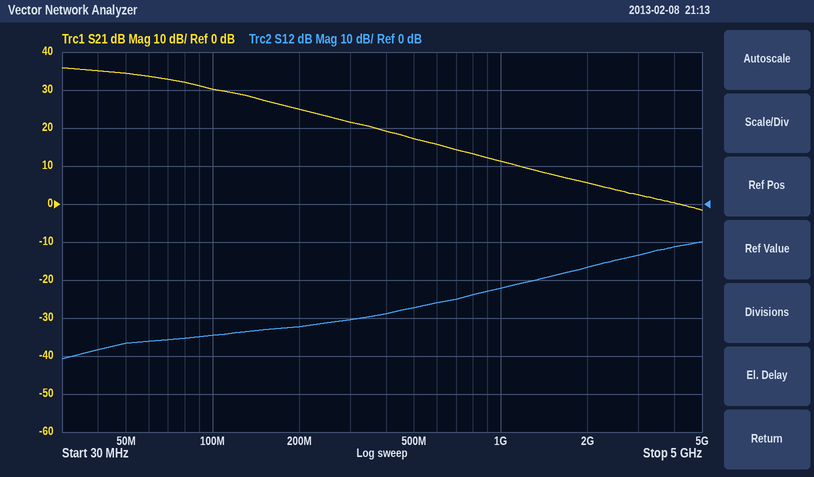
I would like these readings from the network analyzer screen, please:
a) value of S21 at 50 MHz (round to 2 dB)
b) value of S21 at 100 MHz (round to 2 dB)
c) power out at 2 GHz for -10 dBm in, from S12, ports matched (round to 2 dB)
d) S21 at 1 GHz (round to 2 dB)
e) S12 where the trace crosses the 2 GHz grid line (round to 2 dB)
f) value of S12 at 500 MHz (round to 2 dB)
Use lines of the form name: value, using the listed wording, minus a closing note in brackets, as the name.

value of S21 at 50 MHz: 34 dB
value of S21 at 100 MHz: 30 dB
power out at 2 GHz for -10 dBm in, from S12, ports matched: -26 dBm
S21 at 1 GHz: 12 dB
S12 where the trace crosses the 2 GHz grid line: -16 dB
value of S12 at 500 MHz: -28 dB
